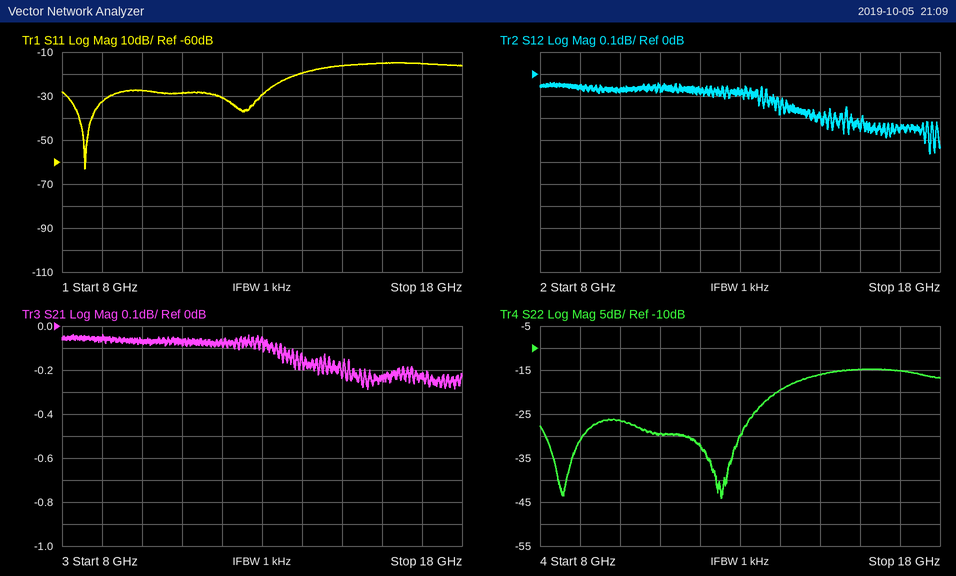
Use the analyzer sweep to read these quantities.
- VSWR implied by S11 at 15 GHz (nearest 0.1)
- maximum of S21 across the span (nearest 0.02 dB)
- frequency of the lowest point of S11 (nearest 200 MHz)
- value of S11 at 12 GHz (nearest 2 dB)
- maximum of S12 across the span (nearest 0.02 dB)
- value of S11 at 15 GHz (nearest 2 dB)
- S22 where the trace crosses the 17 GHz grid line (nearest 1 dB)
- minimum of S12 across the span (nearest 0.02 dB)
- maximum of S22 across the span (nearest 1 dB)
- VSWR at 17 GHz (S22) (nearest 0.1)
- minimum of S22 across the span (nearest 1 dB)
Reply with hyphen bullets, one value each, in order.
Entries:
- 1.4
- -0.04 dB
- 8.6 GHz
- -30 dB
- -0.04 dB
- -16 dB
- -15 dB
- -0.36 dB
- -15 dB
- 1.4
- -44 dB
